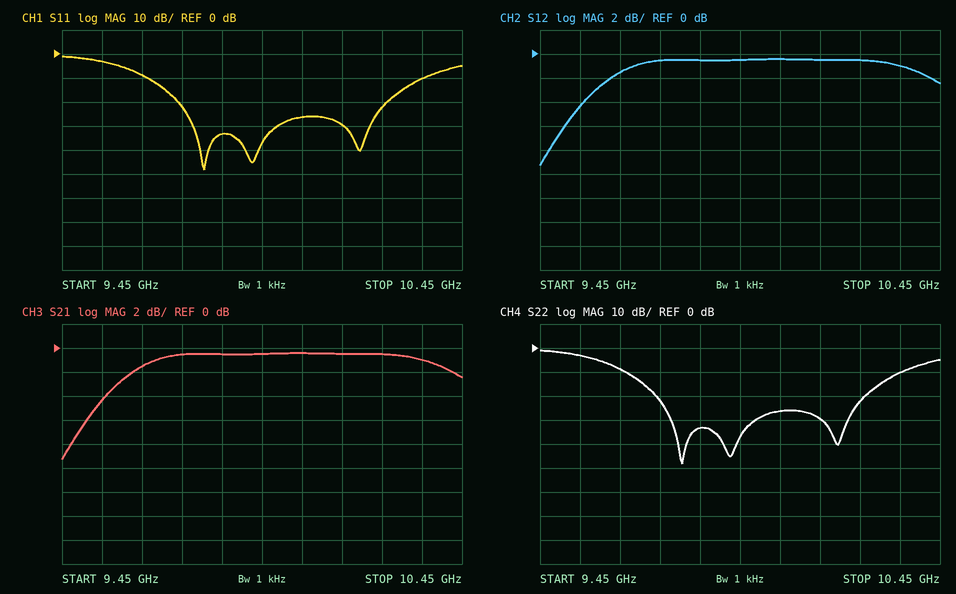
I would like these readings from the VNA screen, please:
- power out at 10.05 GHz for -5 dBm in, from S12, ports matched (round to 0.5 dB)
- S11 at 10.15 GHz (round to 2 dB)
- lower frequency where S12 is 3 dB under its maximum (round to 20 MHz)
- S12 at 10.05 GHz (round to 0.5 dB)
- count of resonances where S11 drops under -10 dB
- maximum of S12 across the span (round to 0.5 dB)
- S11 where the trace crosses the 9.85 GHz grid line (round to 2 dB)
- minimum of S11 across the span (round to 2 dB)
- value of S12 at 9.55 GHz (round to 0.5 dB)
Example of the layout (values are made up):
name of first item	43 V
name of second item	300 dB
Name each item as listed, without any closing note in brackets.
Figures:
power out at 10.05 GHz for -5 dBm in, from S12, ports matched	-5.5 dBm
S11 at 10.15 GHz	-30 dB
lower frequency where S12 is 3 dB under its maximum	9.58 GHz
S12 at 10.05 GHz	-0.5 dB
count of resonances where S11 drops under -10 dB	3
maximum of S12 across the span	-0.5 dB
S11 where the trace crosses the 9.85 GHz grid line	-34 dB
minimum of S11 across the span	-48 dB
value of S12 at 9.55 GHz	-4.5 dB
